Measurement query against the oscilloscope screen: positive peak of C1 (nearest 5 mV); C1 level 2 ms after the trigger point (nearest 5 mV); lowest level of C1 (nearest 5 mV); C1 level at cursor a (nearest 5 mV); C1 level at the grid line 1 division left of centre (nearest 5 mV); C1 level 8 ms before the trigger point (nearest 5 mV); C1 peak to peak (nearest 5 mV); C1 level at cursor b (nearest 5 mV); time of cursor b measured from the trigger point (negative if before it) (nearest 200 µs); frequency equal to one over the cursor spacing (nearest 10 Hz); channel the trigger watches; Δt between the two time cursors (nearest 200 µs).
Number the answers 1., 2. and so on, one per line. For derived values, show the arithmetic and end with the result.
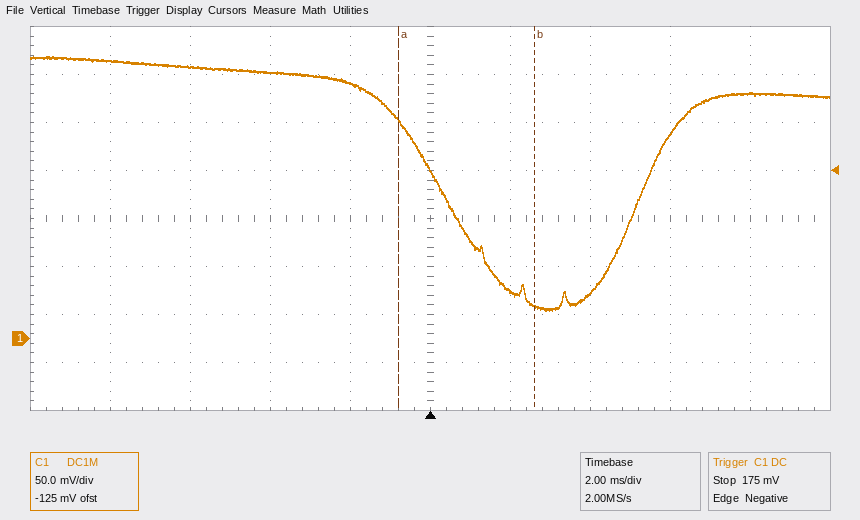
1. 295 mV
2. 50 mV
3. 30 mV
4. 225 mV
5. 265 mV
6. 290 mV
7. 295 mV − (30 mV) = 265 mV
8. 35 mV
9. +2.6 ms
10. 1 / 3.4 ms ≈ 290 Hz
11. C1
12. 3.4 ms
